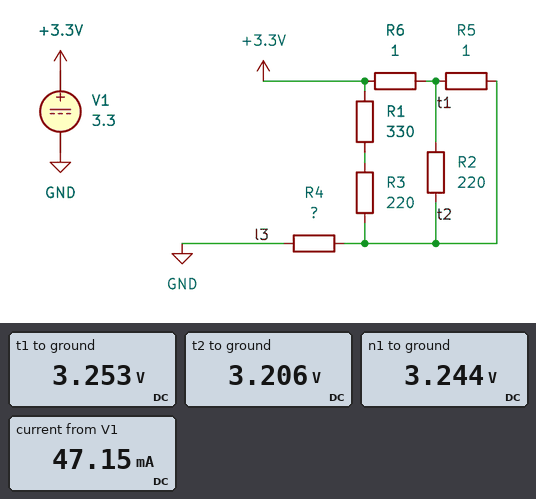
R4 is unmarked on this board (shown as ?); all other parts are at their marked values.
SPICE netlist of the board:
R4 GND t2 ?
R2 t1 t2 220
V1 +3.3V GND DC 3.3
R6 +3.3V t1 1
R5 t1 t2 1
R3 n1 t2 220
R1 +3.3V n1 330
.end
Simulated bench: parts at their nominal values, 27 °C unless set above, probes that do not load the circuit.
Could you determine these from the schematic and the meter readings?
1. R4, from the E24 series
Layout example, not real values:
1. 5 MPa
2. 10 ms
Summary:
1. 68 Ω
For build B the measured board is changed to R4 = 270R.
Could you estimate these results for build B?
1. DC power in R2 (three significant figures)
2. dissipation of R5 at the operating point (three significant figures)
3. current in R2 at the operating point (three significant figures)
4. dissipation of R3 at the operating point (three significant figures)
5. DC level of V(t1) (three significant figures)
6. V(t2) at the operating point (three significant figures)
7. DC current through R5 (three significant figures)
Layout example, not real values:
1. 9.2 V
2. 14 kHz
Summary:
1. 658 nW
2. 145 µW
3. 54.7 µA
4. 423 nW
5. 3.29 V
6. 3.28 V
7. 12.0 mA
